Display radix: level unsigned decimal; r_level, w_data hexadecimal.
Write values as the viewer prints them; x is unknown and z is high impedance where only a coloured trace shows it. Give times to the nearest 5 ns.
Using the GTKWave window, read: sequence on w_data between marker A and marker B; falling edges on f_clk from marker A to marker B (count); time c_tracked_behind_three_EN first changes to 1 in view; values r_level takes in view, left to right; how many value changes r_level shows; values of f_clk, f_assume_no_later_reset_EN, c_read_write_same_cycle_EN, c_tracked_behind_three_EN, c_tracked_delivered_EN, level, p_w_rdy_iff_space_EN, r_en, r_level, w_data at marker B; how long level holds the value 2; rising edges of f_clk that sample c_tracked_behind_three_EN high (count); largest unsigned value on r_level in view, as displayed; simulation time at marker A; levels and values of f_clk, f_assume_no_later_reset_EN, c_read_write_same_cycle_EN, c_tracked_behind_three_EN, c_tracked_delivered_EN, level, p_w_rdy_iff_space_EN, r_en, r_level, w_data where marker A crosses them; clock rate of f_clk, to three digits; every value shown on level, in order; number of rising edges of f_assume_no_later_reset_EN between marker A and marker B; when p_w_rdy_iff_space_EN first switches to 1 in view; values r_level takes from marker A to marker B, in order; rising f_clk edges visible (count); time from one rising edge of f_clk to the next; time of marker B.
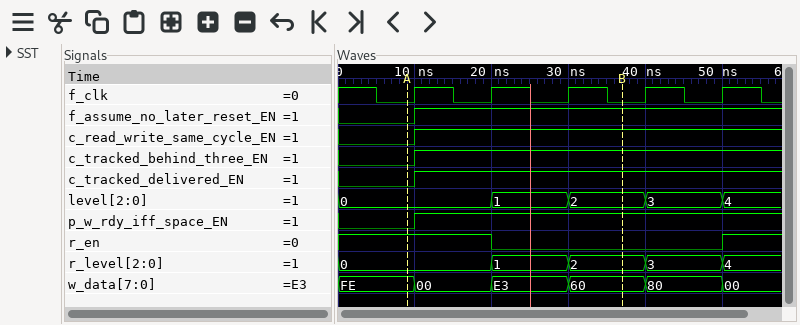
FE, 00, E3, 60
3
10 ns
0, 1, 2, 3, 4
4
f_clk=0, f_assume_no_later_reset_EN=1, c_read_write_same_cycle_EN=1, c_tracked_behind_three_EN=1, c_tracked_delivered_EN=1, level=2, p_w_rdy_iff_space_EN=1, r_en=0, r_level=2, w_data=60
10 ns
4
4
10 ns
f_clk=0, f_assume_no_later_reset_EN=0, c_read_write_same_cycle_EN=0, c_tracked_behind_three_EN=0, c_tracked_delivered_EN=0, level=0, p_w_rdy_iff_space_EN=0, r_en=1, r_level=0, w_data=FE
100 MHz
0, 1, 2, 3, 4
1
10 ns
0, 1, 2
5
10 ns
35 ns
